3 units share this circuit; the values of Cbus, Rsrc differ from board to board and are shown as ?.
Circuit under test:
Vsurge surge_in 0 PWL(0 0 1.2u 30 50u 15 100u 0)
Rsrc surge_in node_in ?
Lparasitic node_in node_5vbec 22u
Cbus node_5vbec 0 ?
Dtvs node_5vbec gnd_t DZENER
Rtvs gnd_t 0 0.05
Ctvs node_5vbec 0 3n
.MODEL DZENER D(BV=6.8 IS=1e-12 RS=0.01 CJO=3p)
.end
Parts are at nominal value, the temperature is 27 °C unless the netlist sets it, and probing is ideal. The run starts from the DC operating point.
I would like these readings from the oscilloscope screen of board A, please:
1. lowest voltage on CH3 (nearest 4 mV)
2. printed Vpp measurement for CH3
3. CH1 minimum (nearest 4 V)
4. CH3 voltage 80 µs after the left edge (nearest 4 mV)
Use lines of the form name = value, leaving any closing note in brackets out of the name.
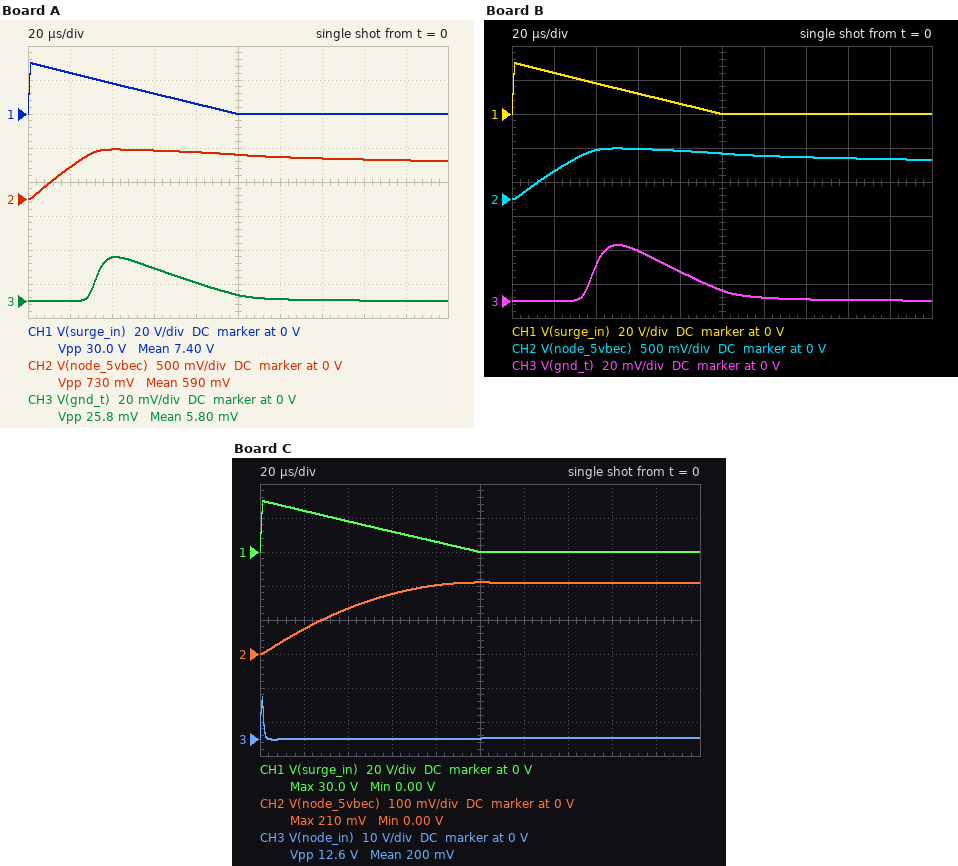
lowest voltage on CH3 = 0 V
printed Vpp measurement for CH3 = 25.8 mV
CH1 minimum = 0 V
CH3 voltage 80 µs after the left edge = 12 mV
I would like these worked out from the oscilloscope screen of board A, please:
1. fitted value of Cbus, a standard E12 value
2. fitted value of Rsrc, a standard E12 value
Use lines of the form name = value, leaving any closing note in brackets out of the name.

fitted value of Cbus, a standard E12 value = 33 µF
fitted value of Rsrc, a standard E12 value = 33 Ω
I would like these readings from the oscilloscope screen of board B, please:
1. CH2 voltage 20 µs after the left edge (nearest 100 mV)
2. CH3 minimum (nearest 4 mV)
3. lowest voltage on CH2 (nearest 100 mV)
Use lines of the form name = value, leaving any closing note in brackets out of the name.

CH2 voltage 20 µs after the left edge = 400 mV
CH3 minimum = 0 V
lowest voltage on CH2 = 0 V
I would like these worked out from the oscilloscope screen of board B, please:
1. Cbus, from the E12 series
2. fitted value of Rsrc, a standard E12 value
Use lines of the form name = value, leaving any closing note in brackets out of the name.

Cbus, from the E12 series = 56 µF
fitted value of Rsrc, a standard E12 value = 22 Ω
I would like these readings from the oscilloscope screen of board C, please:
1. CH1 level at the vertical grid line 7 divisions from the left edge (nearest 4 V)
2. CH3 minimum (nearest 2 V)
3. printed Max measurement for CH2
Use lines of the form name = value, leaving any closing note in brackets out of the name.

CH1 level at the vertical grid line 7 divisions from the left edge = 0 V
CH3 minimum = 0 V
printed Max measurement for CH2 = 210 mV
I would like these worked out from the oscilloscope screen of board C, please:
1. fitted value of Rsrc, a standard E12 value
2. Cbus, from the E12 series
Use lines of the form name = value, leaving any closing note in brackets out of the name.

fitted value of Rsrc, a standard E12 value = 39 Ω
Cbus, from the E12 series = 180 µF
